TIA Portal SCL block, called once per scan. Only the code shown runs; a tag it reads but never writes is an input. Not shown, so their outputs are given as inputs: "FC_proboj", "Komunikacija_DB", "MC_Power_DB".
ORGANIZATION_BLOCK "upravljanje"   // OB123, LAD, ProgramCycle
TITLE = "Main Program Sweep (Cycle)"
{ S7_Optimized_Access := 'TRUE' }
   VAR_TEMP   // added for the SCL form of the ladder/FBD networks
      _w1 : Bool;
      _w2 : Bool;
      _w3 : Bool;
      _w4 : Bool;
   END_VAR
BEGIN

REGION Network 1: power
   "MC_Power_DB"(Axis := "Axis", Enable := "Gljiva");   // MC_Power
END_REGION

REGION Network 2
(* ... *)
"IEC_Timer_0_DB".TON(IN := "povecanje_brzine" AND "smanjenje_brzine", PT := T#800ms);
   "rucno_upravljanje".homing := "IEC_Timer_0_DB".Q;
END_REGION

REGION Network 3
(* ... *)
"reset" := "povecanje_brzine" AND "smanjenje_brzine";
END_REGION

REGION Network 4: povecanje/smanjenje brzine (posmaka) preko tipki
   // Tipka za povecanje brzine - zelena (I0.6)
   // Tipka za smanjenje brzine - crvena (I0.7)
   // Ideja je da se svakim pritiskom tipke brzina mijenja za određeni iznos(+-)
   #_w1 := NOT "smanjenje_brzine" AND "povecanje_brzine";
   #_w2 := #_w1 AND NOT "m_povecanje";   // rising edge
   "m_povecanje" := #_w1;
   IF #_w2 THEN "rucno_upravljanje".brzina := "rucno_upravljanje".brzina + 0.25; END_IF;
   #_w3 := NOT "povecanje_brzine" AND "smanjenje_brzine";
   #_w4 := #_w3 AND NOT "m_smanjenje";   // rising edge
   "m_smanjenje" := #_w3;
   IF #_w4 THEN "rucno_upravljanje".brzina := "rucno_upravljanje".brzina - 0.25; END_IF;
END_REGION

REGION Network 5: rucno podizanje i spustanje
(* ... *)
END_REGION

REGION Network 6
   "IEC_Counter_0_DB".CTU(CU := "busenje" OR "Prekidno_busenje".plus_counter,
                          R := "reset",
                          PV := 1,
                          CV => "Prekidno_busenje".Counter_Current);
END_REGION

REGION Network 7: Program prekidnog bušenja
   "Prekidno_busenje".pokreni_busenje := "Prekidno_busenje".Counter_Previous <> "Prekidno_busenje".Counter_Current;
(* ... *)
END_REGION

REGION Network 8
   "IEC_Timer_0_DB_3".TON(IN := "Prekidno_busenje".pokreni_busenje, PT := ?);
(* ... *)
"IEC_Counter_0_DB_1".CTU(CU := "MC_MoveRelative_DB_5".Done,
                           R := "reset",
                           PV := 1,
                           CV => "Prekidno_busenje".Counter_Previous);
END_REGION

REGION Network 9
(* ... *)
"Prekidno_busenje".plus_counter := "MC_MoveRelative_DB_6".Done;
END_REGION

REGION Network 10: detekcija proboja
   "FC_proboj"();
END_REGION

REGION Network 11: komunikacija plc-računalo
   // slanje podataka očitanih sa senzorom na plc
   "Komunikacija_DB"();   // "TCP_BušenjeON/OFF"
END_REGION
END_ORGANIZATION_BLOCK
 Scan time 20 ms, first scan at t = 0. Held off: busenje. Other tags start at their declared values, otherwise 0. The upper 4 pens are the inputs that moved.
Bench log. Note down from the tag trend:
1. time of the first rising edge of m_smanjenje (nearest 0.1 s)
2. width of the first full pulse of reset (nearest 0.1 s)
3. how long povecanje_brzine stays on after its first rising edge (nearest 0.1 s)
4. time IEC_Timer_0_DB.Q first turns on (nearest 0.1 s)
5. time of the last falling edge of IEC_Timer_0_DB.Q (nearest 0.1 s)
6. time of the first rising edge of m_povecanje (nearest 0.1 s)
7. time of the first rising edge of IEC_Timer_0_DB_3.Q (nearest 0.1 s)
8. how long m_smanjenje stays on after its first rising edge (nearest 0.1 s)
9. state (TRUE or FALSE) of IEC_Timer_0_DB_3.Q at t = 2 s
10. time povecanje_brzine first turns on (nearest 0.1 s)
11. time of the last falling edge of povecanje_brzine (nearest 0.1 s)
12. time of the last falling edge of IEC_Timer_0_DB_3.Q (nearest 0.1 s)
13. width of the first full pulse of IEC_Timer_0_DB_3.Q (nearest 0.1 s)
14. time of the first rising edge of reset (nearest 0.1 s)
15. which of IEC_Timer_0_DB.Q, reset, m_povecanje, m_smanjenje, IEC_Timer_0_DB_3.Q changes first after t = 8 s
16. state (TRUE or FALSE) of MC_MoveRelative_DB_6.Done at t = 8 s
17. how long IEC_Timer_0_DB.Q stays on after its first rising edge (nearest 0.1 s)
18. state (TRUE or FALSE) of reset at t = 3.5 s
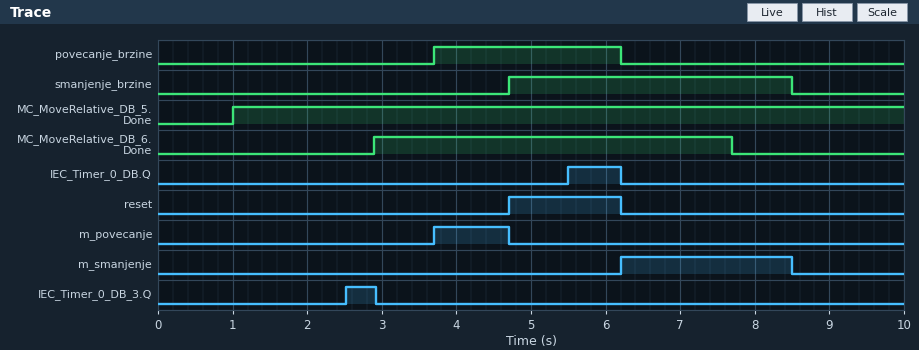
6.2 s
1.5 s
2.5 s
5.5 s
6.2 s
3.7 s
2.5 s
2.3 s
FALSE
3.7 s
6.2 s
2.9 s
0.4 s
4.7 s
m_smanjenje
FALSE
0.7 s
FALSE
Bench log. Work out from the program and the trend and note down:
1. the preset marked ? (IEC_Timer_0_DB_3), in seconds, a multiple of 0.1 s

1.5 s
